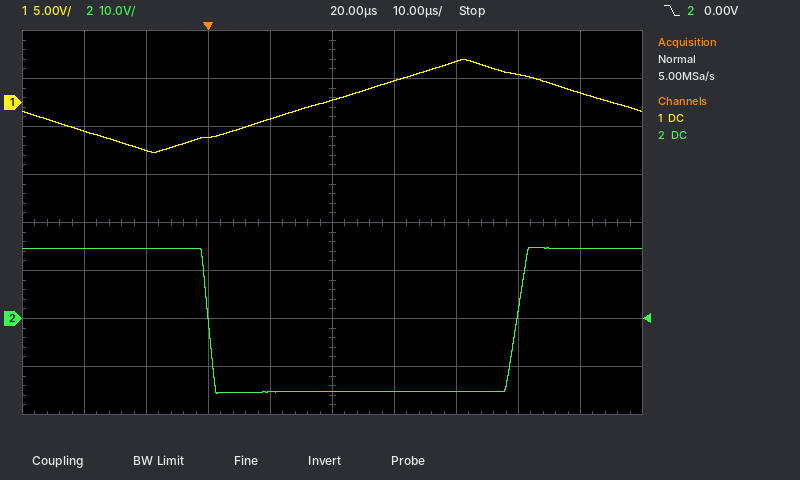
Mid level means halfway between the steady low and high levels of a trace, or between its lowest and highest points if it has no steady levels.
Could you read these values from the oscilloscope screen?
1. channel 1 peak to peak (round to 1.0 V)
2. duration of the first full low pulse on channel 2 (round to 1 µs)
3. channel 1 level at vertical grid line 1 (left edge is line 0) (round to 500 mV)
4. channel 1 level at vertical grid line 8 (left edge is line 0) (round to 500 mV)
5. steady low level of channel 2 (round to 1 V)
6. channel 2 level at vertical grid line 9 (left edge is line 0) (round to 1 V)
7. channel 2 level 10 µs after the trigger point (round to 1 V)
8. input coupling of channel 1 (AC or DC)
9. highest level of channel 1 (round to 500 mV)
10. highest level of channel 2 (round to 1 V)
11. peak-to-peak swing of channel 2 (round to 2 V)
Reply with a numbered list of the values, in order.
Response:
1. 10.0 V
2. 50 µs
3. -3.0 V
4. 3.0 V
5. -15 V
6. 15 V
7. -15 V
8. DC
9. 4.5 V
10. 15 V
11. 30 V
